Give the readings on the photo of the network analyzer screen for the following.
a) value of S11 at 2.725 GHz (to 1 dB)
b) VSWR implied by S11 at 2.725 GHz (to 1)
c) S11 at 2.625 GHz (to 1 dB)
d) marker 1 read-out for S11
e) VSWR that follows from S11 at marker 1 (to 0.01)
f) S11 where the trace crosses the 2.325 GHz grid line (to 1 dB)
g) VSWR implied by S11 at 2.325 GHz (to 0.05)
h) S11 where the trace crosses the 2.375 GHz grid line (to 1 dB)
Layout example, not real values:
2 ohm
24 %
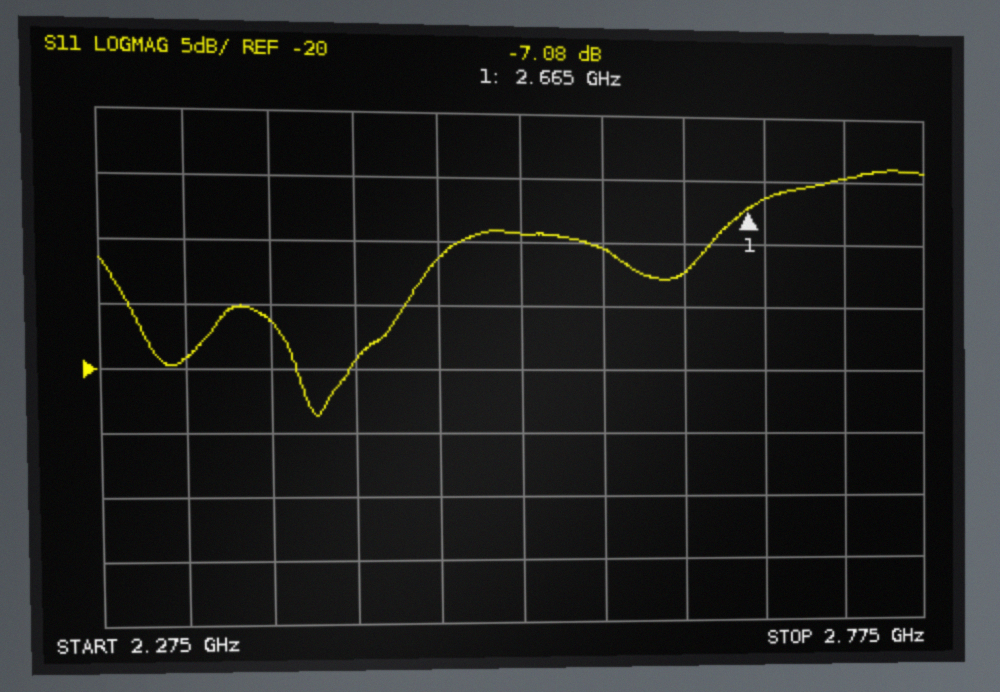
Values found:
-5 dB
4
-12 dB
-7.08 dB
2.59
-19 dB
1.25
-16 dB
